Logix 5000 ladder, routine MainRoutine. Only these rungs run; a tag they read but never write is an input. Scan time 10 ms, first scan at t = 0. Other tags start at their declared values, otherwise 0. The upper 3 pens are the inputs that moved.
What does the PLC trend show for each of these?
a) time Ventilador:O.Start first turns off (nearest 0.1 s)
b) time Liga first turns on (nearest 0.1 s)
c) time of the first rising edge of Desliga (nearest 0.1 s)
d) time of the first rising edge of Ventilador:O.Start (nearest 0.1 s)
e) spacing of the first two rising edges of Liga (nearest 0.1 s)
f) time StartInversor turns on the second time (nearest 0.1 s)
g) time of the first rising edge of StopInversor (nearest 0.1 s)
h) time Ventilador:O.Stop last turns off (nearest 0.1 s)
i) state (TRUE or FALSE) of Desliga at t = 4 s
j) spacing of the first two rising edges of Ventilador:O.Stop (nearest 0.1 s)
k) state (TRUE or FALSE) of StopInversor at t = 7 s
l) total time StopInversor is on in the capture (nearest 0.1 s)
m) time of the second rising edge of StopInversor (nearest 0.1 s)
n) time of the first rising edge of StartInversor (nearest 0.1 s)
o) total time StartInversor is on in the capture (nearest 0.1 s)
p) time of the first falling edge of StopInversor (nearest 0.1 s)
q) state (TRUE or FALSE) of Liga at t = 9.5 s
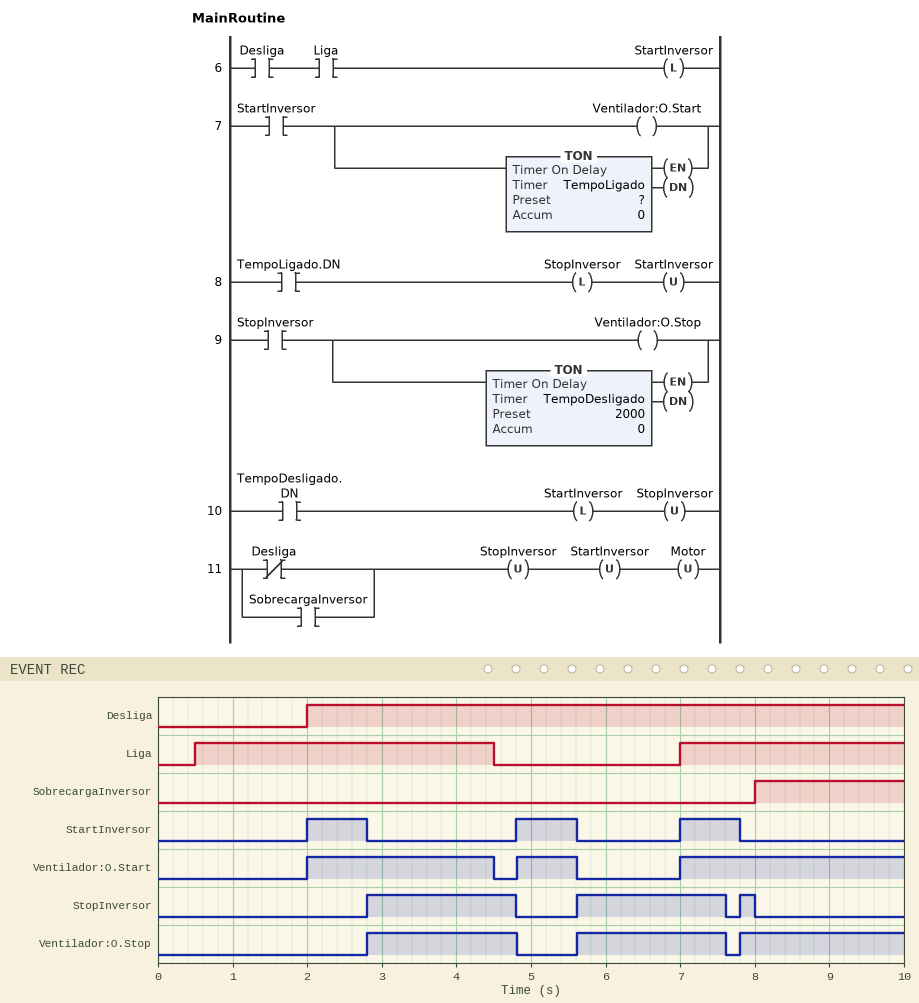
4.5 s
0.5 s
2.0 s
2.0 s
6.5 s
4.8 s
2.8 s
7.6 s
TRUE
2.8 s
TRUE
4.2 s
5.6 s
2.0 s
2.4 s
4.8 s
TRUE
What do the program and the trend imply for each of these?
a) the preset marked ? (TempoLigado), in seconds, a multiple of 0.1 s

0.8 s
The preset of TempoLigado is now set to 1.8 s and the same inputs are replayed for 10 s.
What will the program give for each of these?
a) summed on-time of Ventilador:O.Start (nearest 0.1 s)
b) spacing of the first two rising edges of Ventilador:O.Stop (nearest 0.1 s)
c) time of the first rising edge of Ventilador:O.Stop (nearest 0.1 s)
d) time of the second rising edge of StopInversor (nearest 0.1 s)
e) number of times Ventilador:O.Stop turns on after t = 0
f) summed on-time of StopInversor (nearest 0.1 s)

6.7 s
3.8 s
3.8 s
7.6 s
2
2.4 s
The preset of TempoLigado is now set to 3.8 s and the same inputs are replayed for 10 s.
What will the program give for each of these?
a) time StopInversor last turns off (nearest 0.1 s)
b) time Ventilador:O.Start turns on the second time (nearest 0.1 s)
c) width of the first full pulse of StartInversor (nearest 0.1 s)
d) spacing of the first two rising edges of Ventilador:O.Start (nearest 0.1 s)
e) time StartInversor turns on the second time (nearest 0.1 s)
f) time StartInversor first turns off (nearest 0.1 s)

7.8 s
7.0 s
3.8 s
5.0 s
7.0 s
5.8 s
